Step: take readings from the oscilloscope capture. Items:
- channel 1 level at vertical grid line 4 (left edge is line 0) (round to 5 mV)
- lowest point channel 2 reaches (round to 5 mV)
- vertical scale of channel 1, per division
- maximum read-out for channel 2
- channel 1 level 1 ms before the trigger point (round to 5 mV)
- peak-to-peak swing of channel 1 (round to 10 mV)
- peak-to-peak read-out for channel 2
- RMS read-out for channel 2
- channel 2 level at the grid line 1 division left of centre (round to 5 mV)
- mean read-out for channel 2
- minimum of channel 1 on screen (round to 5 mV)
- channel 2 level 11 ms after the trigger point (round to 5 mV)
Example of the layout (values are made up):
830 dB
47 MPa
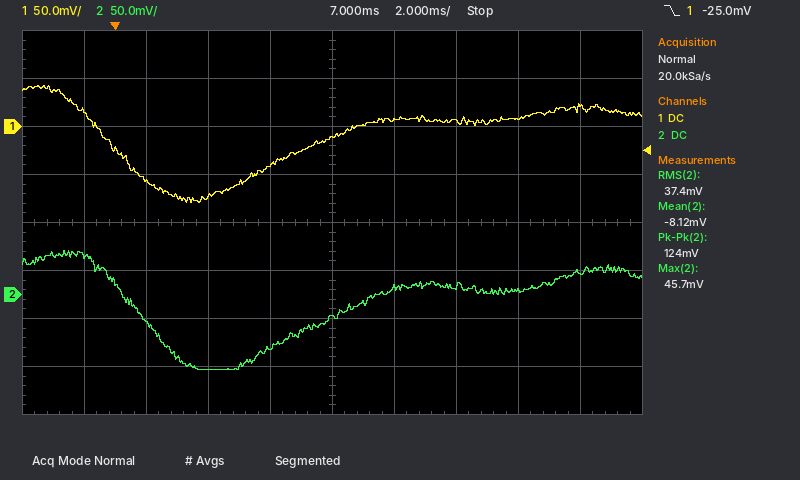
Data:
-40 mV
-80 mV
50 mV
45.7 mV
15 mV
120 mV
124 mV
37.4 mV
-55 mV
-8.12 mV
-80 mV
10 mV
